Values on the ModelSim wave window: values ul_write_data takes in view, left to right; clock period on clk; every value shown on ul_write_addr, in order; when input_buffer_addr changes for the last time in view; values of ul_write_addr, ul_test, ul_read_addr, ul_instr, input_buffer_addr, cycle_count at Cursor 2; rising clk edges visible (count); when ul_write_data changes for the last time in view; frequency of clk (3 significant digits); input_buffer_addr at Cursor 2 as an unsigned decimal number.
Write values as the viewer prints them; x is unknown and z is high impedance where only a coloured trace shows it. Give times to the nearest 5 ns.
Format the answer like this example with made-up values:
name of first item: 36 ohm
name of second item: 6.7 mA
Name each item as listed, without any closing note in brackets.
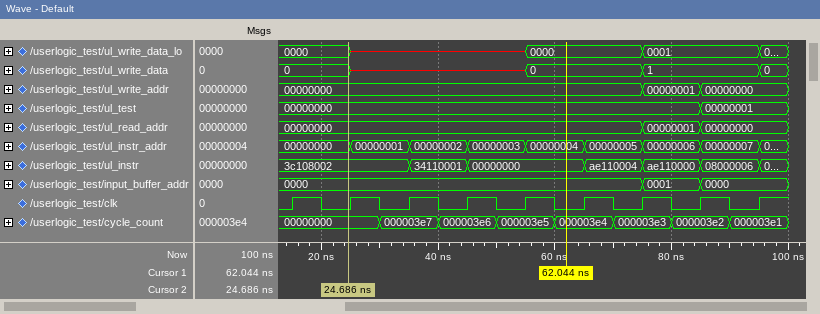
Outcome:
values ul_write_data takes in view, left to right: 0, x, 0, 1, 0
clock period on clk: 10 ns
every value shown on ul_write_addr, in order: 00000000, 00000001, 00000000
when input_buffer_addr changes for the last time in view: 85 ns
values of ul_write_addr, ul_test, ul_read_addr, ul_instr, input_buffer_addr, cycle_count at Cursor 2: ul_write_addr=00000000, ul_test=00000000, ul_read_addr=00000000, ul_instr=3c108002, input_buffer_addr=0000, cycle_count=00000000
rising clk edges visible: 9
when ul_write_data changes for the last time in view: 95 ns
frequency of clk: 100 MHz
input_buffer_addr at Cursor 2 as an unsigned decimal number: 0
